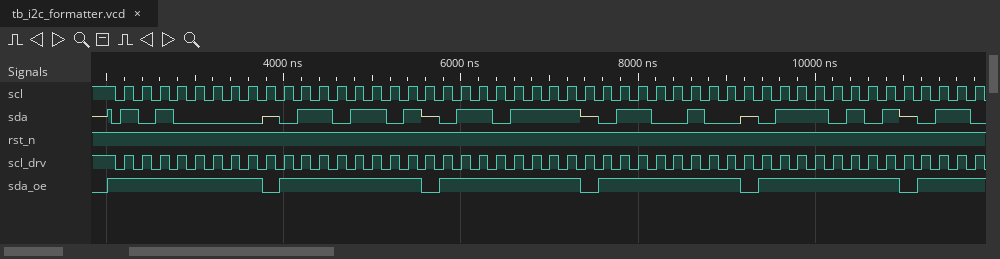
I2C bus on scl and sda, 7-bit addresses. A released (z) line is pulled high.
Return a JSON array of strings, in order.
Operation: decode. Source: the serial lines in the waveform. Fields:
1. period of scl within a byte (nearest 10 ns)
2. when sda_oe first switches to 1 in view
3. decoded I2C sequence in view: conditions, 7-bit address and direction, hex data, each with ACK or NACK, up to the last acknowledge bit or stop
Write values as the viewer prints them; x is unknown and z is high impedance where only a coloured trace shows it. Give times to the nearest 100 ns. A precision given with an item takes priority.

["200 ns", "2000 ns", "start, address 50 write NACK, 6D NACK, 6F NACK, 64 NACK, 75 NACK"]
